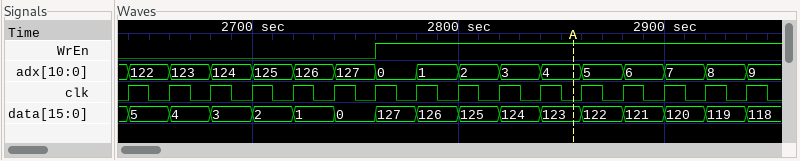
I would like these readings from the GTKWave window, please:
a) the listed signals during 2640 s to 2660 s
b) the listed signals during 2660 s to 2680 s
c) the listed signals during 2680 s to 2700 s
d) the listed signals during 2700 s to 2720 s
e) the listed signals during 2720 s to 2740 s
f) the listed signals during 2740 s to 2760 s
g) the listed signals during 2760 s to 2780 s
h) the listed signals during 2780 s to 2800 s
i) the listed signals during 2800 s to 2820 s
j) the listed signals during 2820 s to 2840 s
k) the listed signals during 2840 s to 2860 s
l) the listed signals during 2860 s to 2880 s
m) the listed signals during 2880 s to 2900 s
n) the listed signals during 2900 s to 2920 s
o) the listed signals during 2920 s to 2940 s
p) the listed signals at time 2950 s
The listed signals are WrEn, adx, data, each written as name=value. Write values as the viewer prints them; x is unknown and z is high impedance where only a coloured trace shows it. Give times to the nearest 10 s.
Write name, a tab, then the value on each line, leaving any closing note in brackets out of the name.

the listed signals during 2640 s to 2660 s	WrEn=0, adx=122, data=5
the listed signals during 2660 s to 2680 s	WrEn=0, adx=123, data=4
the listed signals during 2680 s to 2700 s	WrEn=0, adx=124, data=3
the listed signals during 2700 s to 2720 s	WrEn=0, adx=125, data=2
the listed signals during 2720 s to 2740 s	WrEn=0, adx=126, data=1
the listed signals during 2740 s to 2760 s	WrEn=0, adx=127, data=0
the listed signals during 2760 s to 2780 s	WrEn=1, adx=0, data=127
the listed signals during 2780 s to 2800 s	WrEn=1, adx=1, data=126
the listed signals during 2800 s to 2820 s	WrEn=1, adx=2, data=125
the listed signals during 2820 s to 2840 s	WrEn=1, adx=3, data=124
the listed signals during 2840 s to 2860 s	WrEn=1, adx=4, data=123
the listed signals during 2860 s to 2880 s	WrEn=1, adx=5, data=122
the listed signals during 2880 s to 2900 s	WrEn=1, adx=6, data=121
the listed signals during 2900 s to 2920 s	WrEn=1, adx=7, data=120
the listed signals during 2920 s to 2940 s	WrEn=1, adx=8, data=119
the listed signals at time 2950 s	WrEn=1, adx=9, data=118
